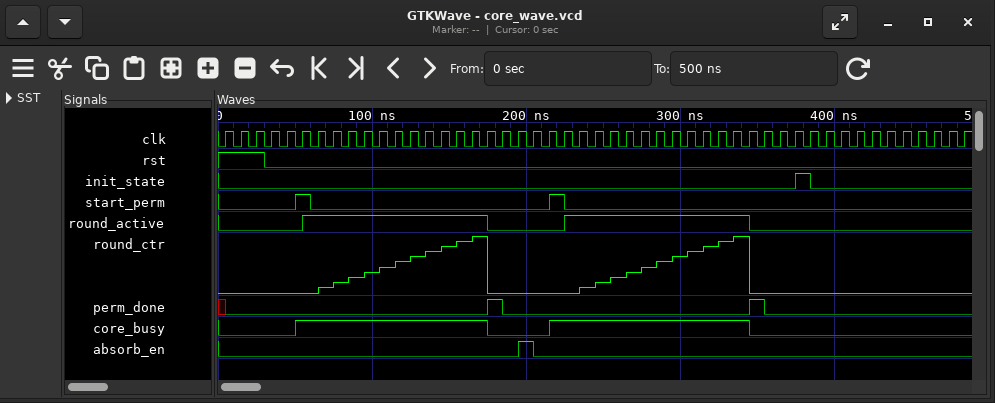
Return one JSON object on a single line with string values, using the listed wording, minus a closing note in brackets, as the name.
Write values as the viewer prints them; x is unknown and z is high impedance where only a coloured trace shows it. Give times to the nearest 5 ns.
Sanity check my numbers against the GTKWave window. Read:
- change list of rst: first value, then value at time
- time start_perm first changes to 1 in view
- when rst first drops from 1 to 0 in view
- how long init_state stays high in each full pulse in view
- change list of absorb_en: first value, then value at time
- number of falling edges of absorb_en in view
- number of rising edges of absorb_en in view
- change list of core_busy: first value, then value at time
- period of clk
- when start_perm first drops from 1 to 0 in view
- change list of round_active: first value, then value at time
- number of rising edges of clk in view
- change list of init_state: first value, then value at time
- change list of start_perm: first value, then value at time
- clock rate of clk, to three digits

{"change list of rst: first value, then value at time": "1, 0 at 30 ns", "time start_perm first changes to 1 in view": "50 ns", "when rst first drops from 1 to 0 in view": "30 ns", "how long init_state stays high in each full pulse in view": "10 ns", "change list of absorb_en: first value, then value at time": "0, 1 at 195 ns, 0 at 205 ns", "number of falling edges of absorb_en in view": "1", "number of rising edges of absorb_en in view": "1", "change list of core_busy: first value, then value at time": "0, 1 at 50 ns, 0 at 175 ns, 1 at 215 ns, 0 at 345 ns", "period of clk": "10 ns", "when start_perm first drops from 1 to 0 in view": "60 ns", "change list of round_active: first value, then value at time": "0, 1 at 55 ns, 0 at 175 ns, 1 at 225 ns, 0 at 345 ns", "number of rising edges of clk in view": "49", "change list of init_state: first value, then value at time": "0, 1 at 375 ns, 0 at 385 ns", "change list of start_perm: first value, then value at time": "0, 1 at 50 ns, 0 at 60 ns, 1 at 215 ns, 0 at 225 ns", "clock rate of clk, to three digits": "100 MHz"}
